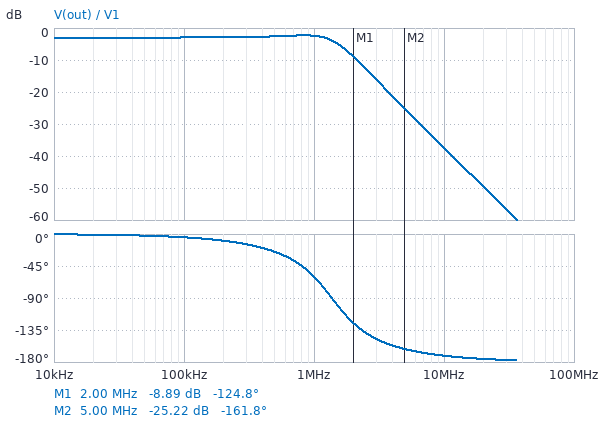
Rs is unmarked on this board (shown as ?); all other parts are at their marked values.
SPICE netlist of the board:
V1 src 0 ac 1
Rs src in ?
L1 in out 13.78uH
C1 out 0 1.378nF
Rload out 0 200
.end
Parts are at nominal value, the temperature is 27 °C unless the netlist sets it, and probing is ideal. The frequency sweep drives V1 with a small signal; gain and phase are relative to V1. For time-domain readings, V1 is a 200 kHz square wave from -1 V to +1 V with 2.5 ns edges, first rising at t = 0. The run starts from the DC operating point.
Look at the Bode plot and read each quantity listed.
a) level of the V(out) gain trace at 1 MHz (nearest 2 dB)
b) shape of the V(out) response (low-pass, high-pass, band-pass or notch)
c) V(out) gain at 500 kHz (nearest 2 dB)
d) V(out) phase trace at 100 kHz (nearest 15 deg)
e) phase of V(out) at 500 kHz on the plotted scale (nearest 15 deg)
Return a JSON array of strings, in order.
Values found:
["-2 dB", "low-pass", "-2 dB", "0 deg", "-30 deg"]
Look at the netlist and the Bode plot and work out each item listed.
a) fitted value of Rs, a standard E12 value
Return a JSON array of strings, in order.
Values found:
["82 Ω"]
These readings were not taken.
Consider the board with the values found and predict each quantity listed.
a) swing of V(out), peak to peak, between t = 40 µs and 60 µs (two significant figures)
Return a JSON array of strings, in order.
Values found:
["1.8 V"]
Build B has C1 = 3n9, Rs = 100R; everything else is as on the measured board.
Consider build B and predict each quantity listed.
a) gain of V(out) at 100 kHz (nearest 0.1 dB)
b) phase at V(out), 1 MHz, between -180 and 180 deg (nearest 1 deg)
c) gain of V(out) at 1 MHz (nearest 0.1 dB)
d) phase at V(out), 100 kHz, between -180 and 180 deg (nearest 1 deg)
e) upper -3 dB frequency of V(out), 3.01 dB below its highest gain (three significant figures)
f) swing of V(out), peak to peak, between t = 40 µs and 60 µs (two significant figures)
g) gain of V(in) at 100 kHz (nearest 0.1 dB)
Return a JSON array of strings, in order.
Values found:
["-3.6 dB", "-102 deg", "-9.4 dB", "-11 deg", "723 kHz", "1.4 V", "-3.7 dB"]
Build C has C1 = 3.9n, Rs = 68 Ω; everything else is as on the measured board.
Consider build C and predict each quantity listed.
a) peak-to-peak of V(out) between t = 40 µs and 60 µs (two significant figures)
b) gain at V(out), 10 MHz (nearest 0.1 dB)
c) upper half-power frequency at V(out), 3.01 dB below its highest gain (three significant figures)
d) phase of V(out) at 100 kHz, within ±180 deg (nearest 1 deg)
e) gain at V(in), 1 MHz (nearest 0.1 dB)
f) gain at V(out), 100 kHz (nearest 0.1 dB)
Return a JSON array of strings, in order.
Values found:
["1.7 V", "-46.5 dB", "870 kHz", "-9 deg", "-5.4 dB", "-2.5 dB"]
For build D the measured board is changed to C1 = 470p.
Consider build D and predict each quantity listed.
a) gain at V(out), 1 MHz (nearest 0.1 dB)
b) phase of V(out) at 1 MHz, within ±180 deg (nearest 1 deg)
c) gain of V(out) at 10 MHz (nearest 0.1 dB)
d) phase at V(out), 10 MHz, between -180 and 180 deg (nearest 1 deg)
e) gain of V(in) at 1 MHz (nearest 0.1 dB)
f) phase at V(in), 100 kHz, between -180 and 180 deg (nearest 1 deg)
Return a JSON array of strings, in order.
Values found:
["-2.5 dB", "-30 deg", "-28.0 dB", "-164 deg", "-3.8 dB", "0 deg"]
